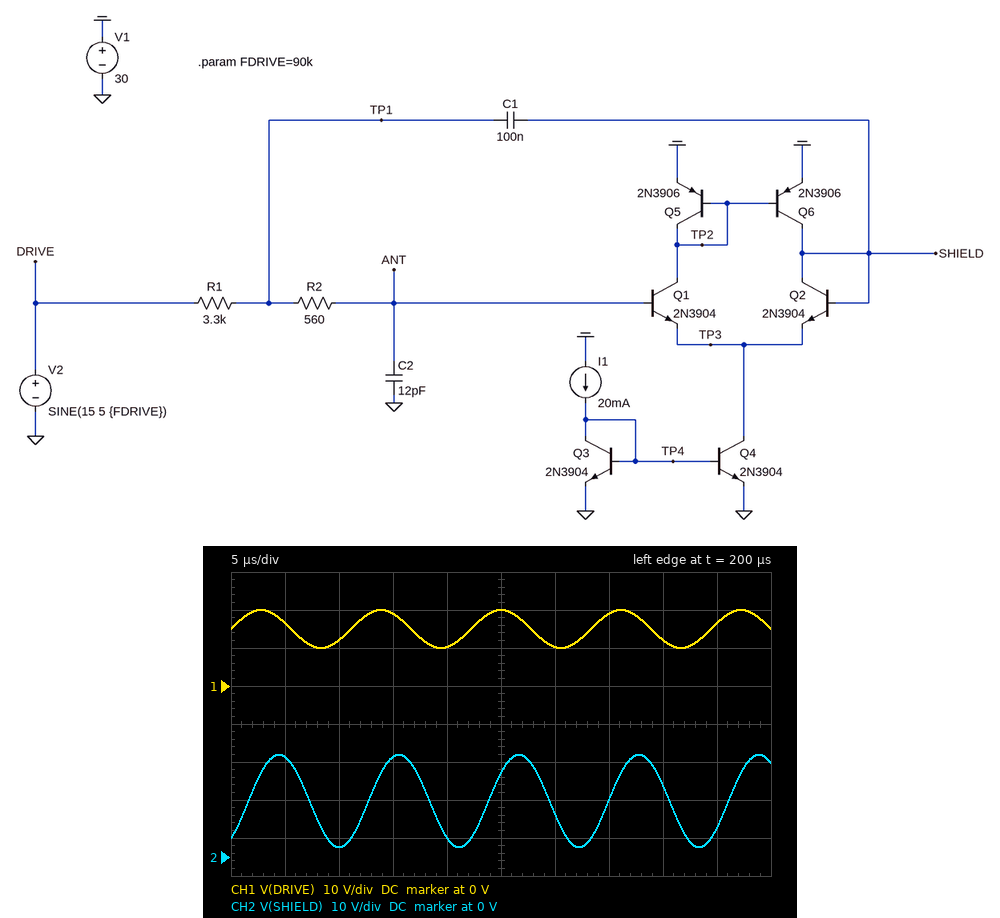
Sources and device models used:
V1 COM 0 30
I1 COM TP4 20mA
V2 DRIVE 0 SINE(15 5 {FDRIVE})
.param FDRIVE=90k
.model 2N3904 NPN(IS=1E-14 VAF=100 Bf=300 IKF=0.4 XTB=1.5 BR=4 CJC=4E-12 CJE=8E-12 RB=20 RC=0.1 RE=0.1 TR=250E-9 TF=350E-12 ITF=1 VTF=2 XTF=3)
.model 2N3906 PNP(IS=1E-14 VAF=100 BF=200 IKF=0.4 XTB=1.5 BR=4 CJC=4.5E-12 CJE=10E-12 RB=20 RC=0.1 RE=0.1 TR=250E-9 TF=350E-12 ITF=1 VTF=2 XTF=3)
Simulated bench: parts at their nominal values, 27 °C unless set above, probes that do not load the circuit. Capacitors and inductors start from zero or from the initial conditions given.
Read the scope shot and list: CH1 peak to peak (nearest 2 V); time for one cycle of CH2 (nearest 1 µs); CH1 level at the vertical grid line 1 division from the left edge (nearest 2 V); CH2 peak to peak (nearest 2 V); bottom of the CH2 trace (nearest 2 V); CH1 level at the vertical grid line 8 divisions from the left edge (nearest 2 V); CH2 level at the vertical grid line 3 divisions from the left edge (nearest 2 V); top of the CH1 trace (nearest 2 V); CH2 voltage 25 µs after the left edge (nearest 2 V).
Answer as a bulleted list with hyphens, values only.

- 10 V
- 11 µs
- 16 V
- 24 V
- 2 V
- 12 V
- 26 V
- 20 V
- 22 V
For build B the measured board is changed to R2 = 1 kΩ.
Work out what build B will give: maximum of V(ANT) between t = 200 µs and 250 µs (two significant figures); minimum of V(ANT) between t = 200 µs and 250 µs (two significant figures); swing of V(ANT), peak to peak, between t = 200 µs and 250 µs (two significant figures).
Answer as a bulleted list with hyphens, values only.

- 23 V
- 7.0 V
- 16 V
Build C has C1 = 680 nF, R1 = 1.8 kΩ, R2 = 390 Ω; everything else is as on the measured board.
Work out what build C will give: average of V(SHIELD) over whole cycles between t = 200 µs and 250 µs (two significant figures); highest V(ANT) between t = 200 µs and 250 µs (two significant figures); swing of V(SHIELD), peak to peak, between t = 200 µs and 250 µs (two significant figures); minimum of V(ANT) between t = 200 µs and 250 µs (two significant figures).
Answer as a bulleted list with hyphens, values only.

- 15 V
- 19 V
- 7.4 V
- 11 V
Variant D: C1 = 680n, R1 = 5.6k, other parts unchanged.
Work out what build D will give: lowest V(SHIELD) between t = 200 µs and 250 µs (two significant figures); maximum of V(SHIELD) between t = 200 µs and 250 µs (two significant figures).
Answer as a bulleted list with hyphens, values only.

- 14 V
- 16 V
